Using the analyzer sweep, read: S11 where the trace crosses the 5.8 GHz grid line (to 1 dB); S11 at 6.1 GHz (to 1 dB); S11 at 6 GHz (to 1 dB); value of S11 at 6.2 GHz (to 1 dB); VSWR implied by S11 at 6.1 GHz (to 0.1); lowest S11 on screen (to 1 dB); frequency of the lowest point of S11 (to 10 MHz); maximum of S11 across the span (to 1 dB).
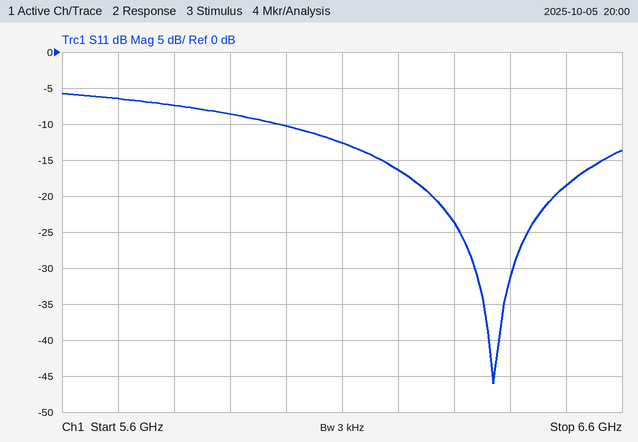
-7 dB
-13 dB
-10 dB
-16 dB
1.6
-46 dB
6.37 GHz
-6 dB
